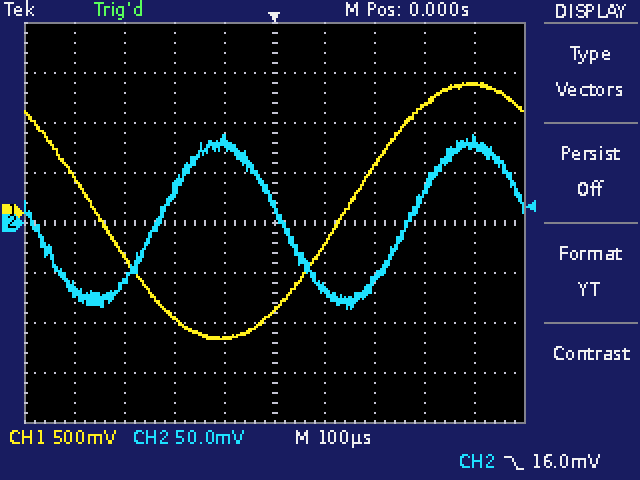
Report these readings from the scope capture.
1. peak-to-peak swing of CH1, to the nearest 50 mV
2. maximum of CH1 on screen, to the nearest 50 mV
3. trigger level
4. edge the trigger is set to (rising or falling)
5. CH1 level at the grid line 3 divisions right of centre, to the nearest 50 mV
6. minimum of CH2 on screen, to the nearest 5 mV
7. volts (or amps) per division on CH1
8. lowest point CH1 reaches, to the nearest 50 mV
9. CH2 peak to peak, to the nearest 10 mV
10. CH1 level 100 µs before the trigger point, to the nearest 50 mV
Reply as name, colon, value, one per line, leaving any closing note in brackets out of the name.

peak-to-peak swing of CH1, to the nearest 50 mV: 2.55 V
maximum of CH1 on screen, to the nearest 50 mV: 1.30 V
trigger level: 16.0 mV
edge the trigger is set to: falling
CH1 level at the grid line 3 divisions right of centre, to the nearest 50 mV: 1.05 V
minimum of CH2 on screen, to the nearest 5 mV: -85 mV
volts (or amps) per division on CH1: 500 mV
lowest point CH1 reaches, to the nearest 50 mV: -1.25 V
CH2 peak to peak, to the nearest 10 mV: 170 mV
CH1 level 100 µs before the trigger point, to the nearest 50 mV: -1.25 V
